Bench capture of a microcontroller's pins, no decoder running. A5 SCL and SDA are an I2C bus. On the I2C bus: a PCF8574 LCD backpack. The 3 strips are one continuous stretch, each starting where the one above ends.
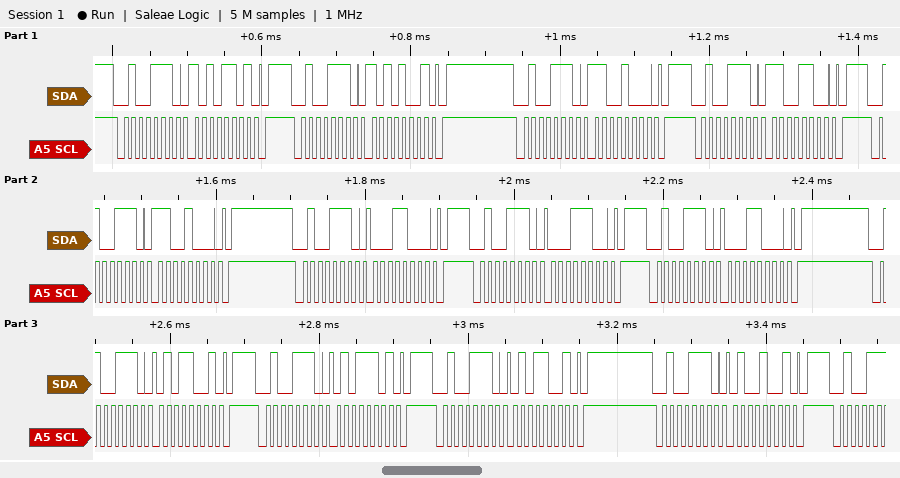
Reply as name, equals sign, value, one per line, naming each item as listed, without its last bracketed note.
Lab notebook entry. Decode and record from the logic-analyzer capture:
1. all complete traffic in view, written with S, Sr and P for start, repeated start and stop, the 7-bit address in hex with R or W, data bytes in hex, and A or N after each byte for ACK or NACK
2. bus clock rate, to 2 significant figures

all complete traffic in view, written with S, Sr and P for start, repeated start and stop, the 7-bit address in hex with R or W, data bytes in hex, and A or N after each byte for ACK or NACK = S 27W A AD A P S 27W A A9 A P S 27W A C8 A P S 27W A CC A P S 27W A C8 A P S 27W A 18 A P S 27W A 1C A P S 27W A 18 A P S 27W A 59 A P S 27W A 5D A P S 27W A 59 A P S 27W A 49 A P
bus clock rate, to 2 significant figures = 100 kHz
